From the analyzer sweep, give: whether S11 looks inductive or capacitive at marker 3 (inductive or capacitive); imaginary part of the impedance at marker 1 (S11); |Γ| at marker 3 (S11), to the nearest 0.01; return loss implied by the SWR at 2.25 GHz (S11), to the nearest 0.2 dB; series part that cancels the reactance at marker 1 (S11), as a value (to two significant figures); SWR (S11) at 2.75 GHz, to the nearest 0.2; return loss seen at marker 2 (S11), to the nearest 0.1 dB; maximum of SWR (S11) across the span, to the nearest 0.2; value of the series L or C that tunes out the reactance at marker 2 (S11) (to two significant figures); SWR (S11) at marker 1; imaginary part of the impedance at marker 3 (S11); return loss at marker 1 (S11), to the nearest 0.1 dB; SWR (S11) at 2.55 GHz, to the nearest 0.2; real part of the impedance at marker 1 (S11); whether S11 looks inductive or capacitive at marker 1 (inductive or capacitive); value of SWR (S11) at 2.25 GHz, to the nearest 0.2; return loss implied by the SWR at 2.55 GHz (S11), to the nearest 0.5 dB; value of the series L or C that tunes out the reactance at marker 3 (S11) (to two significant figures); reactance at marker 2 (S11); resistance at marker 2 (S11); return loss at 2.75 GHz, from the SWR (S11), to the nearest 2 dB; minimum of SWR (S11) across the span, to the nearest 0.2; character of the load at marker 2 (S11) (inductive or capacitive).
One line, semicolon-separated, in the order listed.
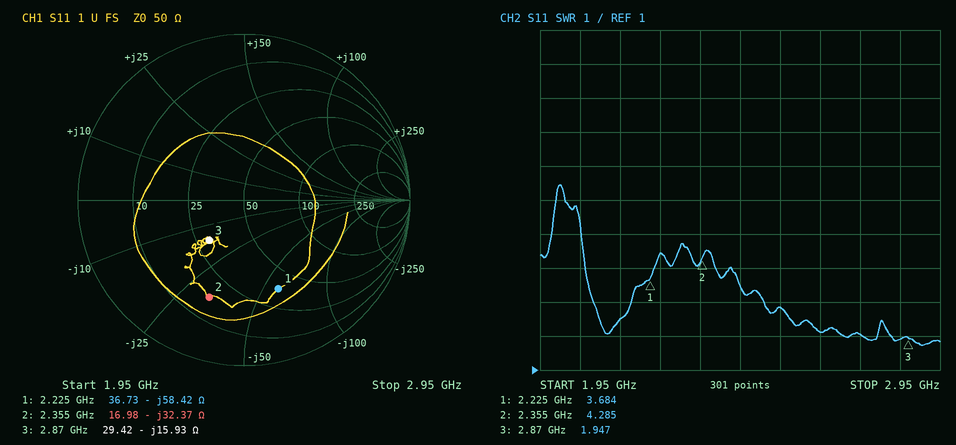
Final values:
capacitive; -58.42 Ω; 0.32; 4.0 dB; 4.2 nH; 2.0; 4.1 dB; 6.4; 2.2 nH; 3.684; -15.93 Ω; 4.8 dB; 2.8; 36.73 Ω; capacitive; 4.4; 6.5 dB; 880 pH; -32.37 Ω; 16.98 Ω; 10 dB; 1.8; capacitive
